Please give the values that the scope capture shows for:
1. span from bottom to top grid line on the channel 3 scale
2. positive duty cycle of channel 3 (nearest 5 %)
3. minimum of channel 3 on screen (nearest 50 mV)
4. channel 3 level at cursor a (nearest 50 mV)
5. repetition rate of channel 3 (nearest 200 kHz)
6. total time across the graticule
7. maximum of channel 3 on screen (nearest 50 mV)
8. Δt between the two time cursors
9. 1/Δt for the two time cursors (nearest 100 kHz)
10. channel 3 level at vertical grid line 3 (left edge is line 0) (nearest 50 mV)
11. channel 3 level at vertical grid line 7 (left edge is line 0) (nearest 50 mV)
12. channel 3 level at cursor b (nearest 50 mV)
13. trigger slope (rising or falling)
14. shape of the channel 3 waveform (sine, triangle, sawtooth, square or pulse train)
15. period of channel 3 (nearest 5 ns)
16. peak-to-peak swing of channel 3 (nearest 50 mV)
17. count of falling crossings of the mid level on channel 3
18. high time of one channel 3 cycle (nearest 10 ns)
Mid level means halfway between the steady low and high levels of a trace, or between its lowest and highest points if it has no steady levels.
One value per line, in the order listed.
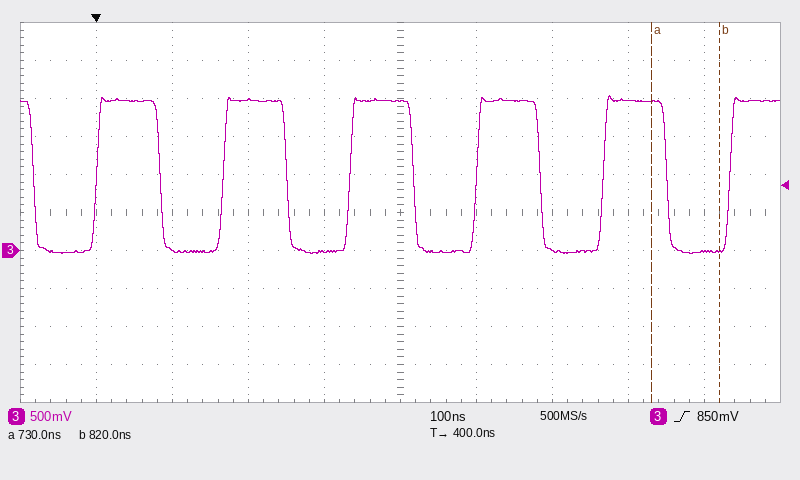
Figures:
5 V
50 %
-50 mV
1.95 V
6.0 MHz
1 µs
2.05 V
90 ns
11.1 MHz
2.00 V
0 mV
0 mV
rising
square
165 ns
2.10 V
6
80 ns
